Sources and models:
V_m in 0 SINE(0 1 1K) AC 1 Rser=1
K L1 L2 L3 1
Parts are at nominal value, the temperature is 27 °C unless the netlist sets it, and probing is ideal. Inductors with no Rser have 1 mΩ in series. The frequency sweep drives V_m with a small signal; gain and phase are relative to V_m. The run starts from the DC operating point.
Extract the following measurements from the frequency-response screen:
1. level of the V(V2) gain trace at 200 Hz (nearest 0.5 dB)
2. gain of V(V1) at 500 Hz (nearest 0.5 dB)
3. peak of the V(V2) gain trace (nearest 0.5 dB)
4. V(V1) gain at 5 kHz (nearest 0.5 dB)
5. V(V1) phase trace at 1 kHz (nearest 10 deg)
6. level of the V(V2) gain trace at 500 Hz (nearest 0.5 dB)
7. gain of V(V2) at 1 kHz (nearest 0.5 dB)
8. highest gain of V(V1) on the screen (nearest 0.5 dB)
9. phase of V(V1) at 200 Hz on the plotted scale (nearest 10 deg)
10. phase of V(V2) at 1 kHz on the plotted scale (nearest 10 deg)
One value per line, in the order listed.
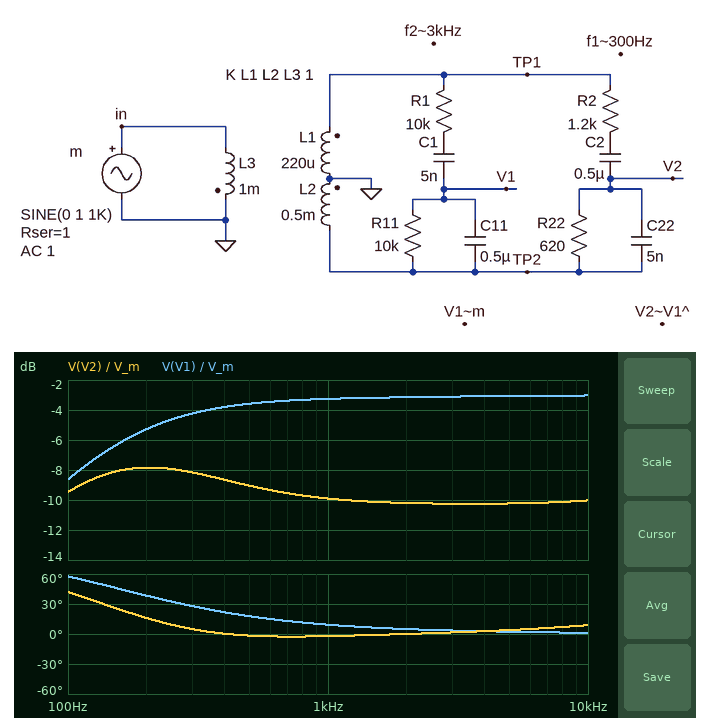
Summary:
-8.0 dB
-3.5 dB
-8.0 dB
-3.0 dB
10 deg
-9.0 dB
-10.0 dB
-3.0 dB
40 deg
0 deg
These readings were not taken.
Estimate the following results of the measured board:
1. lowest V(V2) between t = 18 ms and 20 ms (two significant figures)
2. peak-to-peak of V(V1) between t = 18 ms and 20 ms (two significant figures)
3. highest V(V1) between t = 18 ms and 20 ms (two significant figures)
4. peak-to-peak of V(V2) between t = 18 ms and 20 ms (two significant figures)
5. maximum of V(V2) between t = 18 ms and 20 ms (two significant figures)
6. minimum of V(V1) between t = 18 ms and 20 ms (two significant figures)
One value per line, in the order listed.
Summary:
-320 mV
1.4 V
690 mV
640 mV
320 mV
-690 mV
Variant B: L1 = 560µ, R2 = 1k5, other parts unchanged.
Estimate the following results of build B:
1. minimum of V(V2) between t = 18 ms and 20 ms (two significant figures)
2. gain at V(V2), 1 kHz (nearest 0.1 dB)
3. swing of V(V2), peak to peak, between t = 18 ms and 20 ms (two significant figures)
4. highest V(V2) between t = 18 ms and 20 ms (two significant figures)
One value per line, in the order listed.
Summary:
-290 mV
-10.7 dB
580 mV
290 mV
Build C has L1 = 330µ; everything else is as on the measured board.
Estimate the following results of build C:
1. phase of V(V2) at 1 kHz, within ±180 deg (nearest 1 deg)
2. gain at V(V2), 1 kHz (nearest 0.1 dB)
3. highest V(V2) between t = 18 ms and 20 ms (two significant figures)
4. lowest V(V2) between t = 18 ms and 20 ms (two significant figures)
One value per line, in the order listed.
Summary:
-5 deg
-10.8 dB
290 mV
-290 mV
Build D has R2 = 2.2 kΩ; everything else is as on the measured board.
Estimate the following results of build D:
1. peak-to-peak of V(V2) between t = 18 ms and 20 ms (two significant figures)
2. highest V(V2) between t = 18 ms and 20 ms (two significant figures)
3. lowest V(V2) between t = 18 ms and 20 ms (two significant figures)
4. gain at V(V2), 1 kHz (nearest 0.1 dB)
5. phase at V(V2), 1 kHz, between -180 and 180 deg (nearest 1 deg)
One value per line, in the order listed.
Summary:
890 mV
450 mV
-450 mV
-7.0 dB
6 deg
